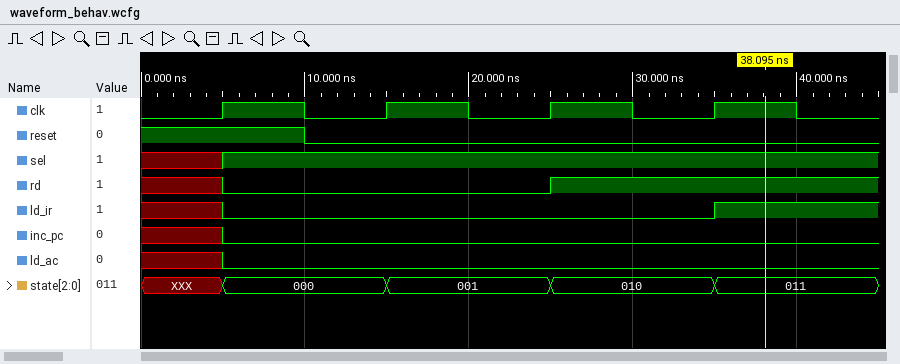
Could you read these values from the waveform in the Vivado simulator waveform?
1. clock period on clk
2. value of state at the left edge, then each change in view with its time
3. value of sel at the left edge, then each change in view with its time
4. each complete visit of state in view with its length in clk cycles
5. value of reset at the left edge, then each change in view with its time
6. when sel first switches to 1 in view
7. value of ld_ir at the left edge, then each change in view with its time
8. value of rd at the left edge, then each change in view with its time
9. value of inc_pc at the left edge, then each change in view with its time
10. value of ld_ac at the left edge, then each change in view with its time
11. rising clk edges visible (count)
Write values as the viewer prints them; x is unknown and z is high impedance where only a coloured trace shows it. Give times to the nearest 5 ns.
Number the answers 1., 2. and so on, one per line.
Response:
1. 10 ns
2. XXX, 000 at 5 ns, 001 at 15 ns, 010 at 25 ns, 011 at 35 ns
3. x, 1 at 5 ns
4. 000: 1, 001: 1, 010: 1
5. 1, 0 at 10 ns
6. 5 ns
7. x, 0 at 5 ns, 1 at 35 ns
8. x, 0 at 5 ns, 1 at 25 ns
9. x, 0 at 5 ns
10. x, 0 at 5 ns
11. 4
